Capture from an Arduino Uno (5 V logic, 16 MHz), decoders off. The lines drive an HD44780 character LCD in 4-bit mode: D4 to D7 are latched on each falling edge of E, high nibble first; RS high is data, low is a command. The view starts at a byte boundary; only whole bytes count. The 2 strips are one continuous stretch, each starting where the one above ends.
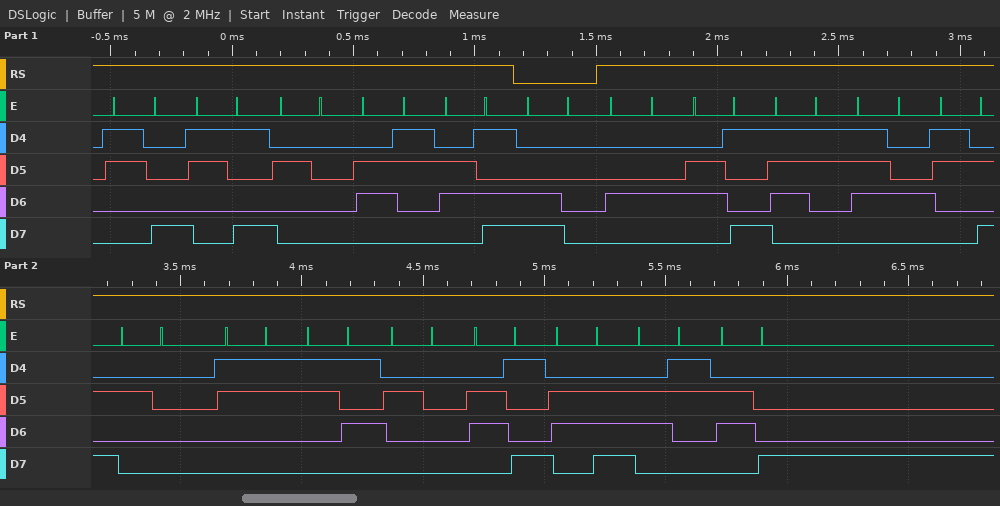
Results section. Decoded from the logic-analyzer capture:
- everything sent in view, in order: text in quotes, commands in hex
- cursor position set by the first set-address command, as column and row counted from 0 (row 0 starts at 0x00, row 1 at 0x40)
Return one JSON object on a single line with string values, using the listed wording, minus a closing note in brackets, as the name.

{"everything sent in view, in order: text in quotes, commands in hex": "\"89 cm\" 0xC0 \"Dist: 35 inch\"", "cursor position set by the first set-address command, as column and row counted from 0": "column 0, row 1"}
